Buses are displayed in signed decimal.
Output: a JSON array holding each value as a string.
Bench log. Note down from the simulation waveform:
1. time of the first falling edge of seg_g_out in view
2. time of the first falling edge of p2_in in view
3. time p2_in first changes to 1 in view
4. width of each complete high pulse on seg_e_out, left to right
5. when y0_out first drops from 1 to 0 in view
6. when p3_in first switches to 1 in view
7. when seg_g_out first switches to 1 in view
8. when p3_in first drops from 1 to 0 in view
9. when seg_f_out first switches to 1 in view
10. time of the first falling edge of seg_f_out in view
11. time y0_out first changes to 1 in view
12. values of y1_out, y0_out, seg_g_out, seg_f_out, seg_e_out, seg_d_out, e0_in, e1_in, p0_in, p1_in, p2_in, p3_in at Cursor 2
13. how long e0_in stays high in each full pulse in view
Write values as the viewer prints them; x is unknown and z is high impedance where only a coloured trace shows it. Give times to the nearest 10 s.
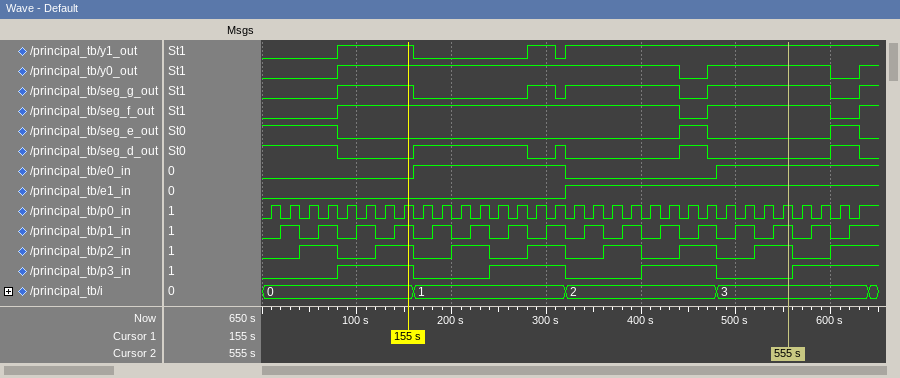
["160 s", "80 s", "40 s", "30 s, 30 s", "440 s", "80 s", "80 s", "160 s", "80 s", "440 s", "80 s", "y1_out=1, y0_out=1, seg_g_out=1, seg_f_out=1, seg_e_out=0, seg_d_out=0, e0_in=1, e1_in=1, p0_in=1, p1_in=1, p2_in=1, p3_in=0", "160 s"]
